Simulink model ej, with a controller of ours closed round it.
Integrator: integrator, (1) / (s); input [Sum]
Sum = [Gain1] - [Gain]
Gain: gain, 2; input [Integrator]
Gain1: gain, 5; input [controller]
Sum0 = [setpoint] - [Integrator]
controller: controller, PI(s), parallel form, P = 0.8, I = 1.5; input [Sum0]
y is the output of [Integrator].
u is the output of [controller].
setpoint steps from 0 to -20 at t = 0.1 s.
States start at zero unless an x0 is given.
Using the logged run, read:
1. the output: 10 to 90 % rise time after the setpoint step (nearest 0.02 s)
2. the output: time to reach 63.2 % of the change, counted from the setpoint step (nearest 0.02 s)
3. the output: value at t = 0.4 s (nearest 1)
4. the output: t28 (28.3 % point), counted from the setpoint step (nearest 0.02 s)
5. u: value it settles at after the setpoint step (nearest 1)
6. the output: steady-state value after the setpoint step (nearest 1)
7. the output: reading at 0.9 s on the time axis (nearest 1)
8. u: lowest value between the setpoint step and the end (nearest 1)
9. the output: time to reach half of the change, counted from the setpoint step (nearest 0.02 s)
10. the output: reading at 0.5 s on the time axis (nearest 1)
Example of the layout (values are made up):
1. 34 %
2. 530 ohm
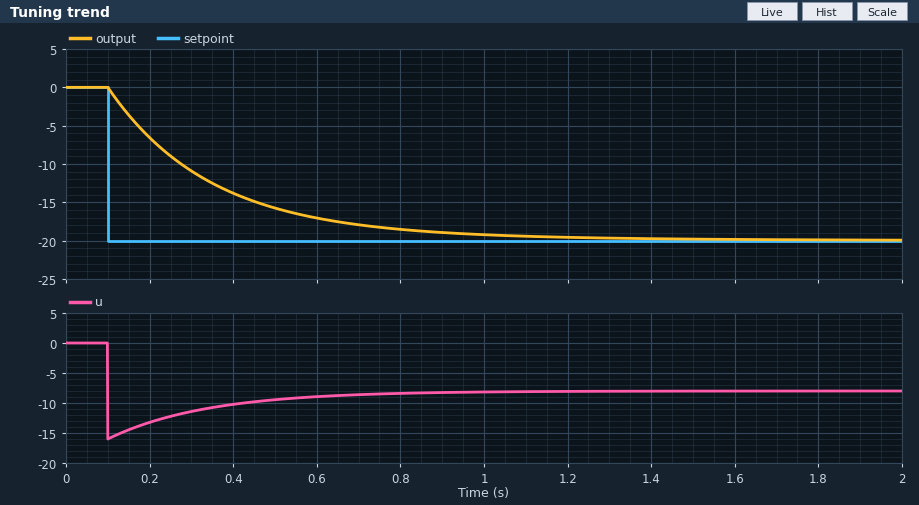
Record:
1. 0.58 s
2. 0.26 s
3. -14
4. 0.08 s
5. -8
6. -20
7. -19
8. -16
9. 0.18 s
10. -16
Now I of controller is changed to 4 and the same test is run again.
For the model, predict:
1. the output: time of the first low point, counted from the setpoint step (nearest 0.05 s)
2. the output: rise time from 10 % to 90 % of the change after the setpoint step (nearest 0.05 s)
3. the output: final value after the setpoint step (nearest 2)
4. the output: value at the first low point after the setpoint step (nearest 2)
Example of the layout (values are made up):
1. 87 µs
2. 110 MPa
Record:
1. 0.65 s
2. 0.30 s
3. -20
4. -22
